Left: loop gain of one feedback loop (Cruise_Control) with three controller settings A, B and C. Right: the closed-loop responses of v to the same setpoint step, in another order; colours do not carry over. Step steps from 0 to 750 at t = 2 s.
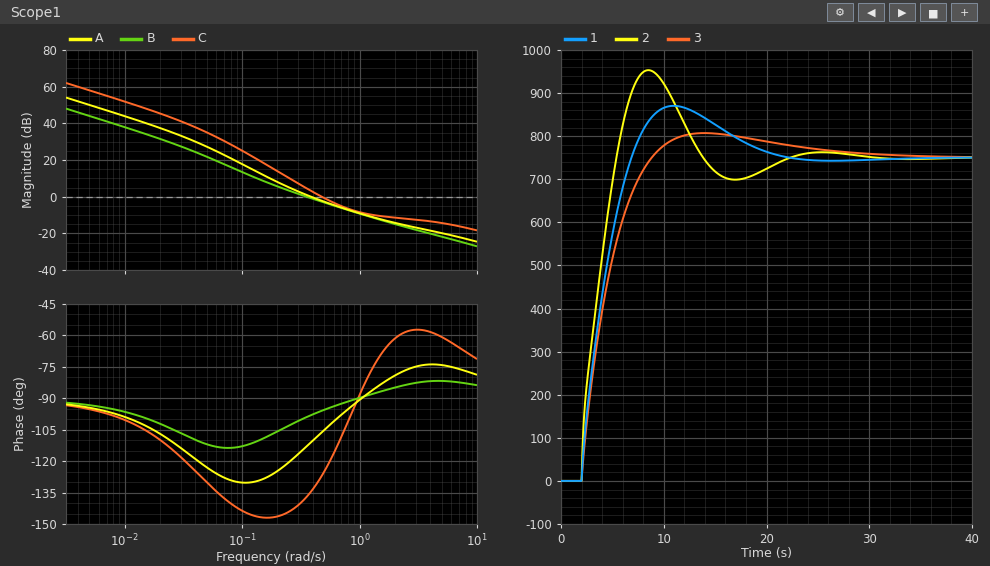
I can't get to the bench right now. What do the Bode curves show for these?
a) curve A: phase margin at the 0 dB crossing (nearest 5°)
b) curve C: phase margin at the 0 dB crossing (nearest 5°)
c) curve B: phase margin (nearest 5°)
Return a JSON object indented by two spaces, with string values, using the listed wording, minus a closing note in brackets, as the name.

{
  "curve A: phase margin at the 0 dB crossing": "70°",
  "curve C: phase margin at the 0 dB crossing": "55°",
  "curve B: phase margin": "80°"
}
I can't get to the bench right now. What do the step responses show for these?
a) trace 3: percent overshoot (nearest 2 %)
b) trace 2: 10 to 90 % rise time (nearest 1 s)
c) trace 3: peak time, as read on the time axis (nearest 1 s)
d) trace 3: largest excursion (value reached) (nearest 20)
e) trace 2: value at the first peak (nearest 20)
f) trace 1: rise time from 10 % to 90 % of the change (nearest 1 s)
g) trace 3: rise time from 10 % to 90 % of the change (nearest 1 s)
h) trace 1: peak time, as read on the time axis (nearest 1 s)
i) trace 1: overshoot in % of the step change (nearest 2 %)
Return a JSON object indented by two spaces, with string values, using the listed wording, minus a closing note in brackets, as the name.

{
  "trace 3: percent overshoot": "8 %",
  "trace 2: 10 to 90 % rise time": "3 s",
  "trace 3: peak time, as read on the time axis": "14 s",
  "trace 3: largest excursion (value reached)": "800",
  "trace 2: value at the first peak": "960",
  "trace 1: rise time from 10 % to 90 % of the change": "4 s",
  "trace 3: rise time from 10 % to 90 % of the change": "5 s",
  "trace 1: peak time, as read on the time axis": "11 s",
  "trace 1: overshoot in % of the step change": "16 %"
}
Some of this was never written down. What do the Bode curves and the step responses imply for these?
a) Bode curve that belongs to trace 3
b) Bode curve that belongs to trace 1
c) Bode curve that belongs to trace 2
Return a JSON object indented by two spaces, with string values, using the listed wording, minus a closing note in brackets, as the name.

{
  "Bode curve that belongs to trace 3": "B",
  "Bode curve that belongs to trace 1": "A",
  "Bode curve that belongs to trace 2": "C"
}
